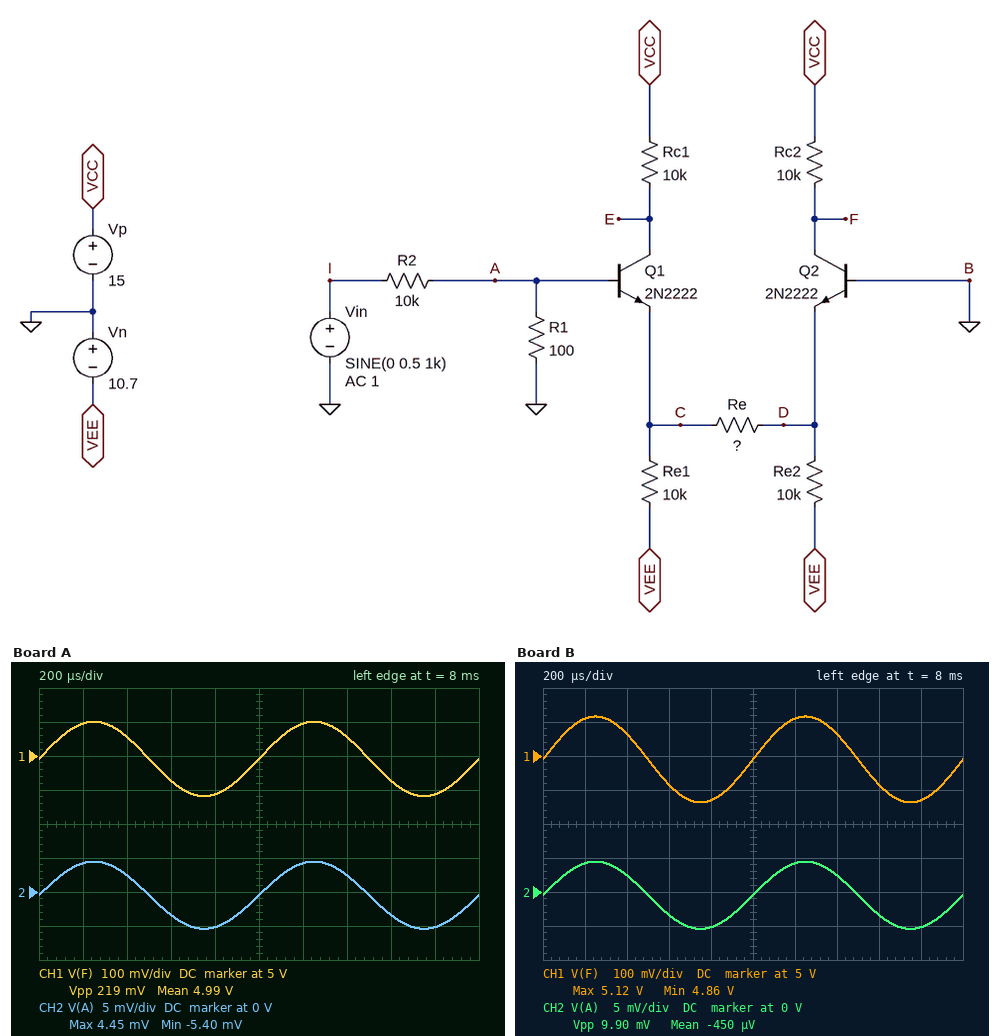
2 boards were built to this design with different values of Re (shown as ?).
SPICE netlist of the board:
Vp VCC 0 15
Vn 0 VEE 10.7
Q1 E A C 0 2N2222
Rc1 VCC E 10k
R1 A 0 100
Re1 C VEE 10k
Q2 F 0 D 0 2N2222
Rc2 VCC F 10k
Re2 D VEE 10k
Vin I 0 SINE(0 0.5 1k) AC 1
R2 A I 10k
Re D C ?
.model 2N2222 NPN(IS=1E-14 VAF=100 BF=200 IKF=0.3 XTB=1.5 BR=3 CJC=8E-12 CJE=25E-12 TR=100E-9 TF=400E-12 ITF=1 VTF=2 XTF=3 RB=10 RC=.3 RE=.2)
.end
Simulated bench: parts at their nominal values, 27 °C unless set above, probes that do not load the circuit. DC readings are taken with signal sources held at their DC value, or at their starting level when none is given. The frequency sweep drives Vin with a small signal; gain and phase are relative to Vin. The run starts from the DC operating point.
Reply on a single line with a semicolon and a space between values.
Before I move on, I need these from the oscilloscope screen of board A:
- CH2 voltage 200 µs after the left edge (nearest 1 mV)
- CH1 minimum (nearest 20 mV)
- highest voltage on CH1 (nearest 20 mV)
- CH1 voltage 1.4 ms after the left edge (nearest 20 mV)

4 mV; 4.88 V; 5.10 V; 5.06 V
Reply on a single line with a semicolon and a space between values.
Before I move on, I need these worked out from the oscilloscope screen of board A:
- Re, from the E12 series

390 Ω
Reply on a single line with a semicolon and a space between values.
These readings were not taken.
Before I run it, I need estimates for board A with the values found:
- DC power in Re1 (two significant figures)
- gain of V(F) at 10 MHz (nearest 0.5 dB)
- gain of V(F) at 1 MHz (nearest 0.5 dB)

10 mW; -24.0 dB; -13.5 dB
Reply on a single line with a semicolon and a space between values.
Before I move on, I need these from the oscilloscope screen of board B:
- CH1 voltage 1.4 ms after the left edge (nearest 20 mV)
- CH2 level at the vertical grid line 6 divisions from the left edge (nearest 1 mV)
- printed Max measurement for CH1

5.06 V; 4 mV; 5.12 V
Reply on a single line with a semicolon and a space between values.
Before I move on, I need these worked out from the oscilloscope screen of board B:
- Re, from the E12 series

330 Ω
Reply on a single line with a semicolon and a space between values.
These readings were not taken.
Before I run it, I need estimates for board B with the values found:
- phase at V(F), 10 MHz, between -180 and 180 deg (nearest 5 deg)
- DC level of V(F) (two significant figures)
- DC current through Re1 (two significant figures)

-80 deg; 5.0 V; 1.0 mA
